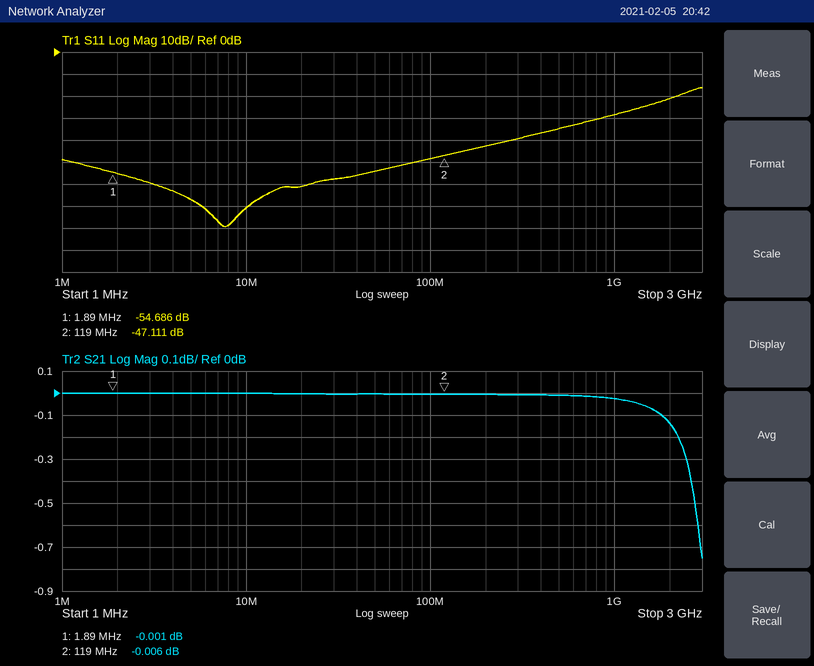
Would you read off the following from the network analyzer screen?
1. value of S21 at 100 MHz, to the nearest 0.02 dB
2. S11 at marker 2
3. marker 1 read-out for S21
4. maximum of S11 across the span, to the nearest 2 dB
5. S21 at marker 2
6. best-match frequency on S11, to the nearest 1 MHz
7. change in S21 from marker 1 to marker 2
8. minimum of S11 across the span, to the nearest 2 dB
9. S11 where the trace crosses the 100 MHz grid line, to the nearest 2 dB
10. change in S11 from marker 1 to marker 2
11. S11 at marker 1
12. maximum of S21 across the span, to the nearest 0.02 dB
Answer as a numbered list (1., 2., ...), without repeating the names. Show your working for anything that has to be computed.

1. 0.00 dB
2. -47.111 dB
3. -0.001 dB
4. -16 dB
5. -0.006 dB
6. 8 MHz
7. -0.006 − (-0.001) = -0.005 dB
8. -80 dB
9. -48 dB
10. -47.111 − (-54.686) = 7.575 dB
11. -54.686 dB
12. 0.00 dB
